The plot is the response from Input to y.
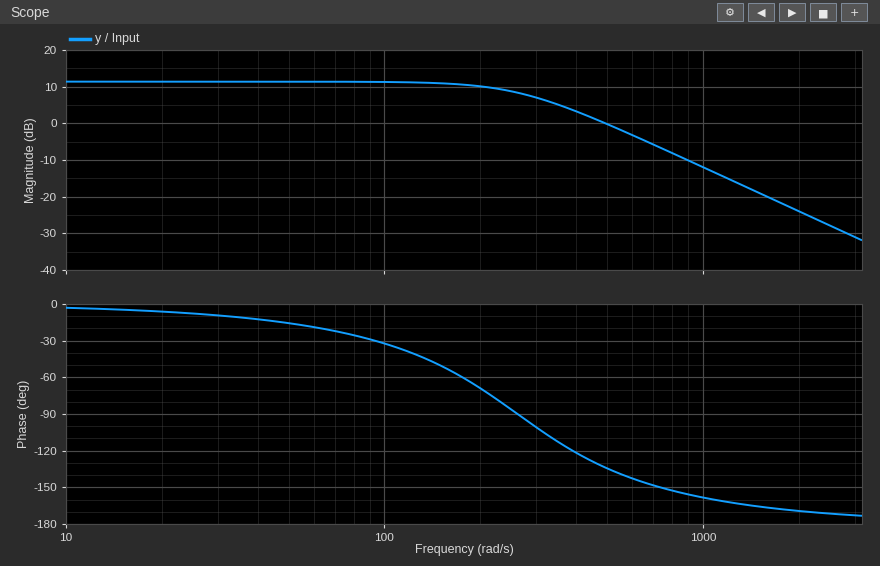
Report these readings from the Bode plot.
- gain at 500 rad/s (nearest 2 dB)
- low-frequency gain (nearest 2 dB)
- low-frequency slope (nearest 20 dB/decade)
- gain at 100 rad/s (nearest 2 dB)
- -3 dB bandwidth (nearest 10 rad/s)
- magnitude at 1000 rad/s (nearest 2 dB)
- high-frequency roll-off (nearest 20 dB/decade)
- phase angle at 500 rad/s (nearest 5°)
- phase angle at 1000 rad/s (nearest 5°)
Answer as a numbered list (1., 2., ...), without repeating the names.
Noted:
1. 0 dB
2. 12 dB
3. 0 dB/decade
4. 12 dB
5. 260 rad/s
6. -12 dB
7. -40 dB/decade
8. -135°
9. -160°
